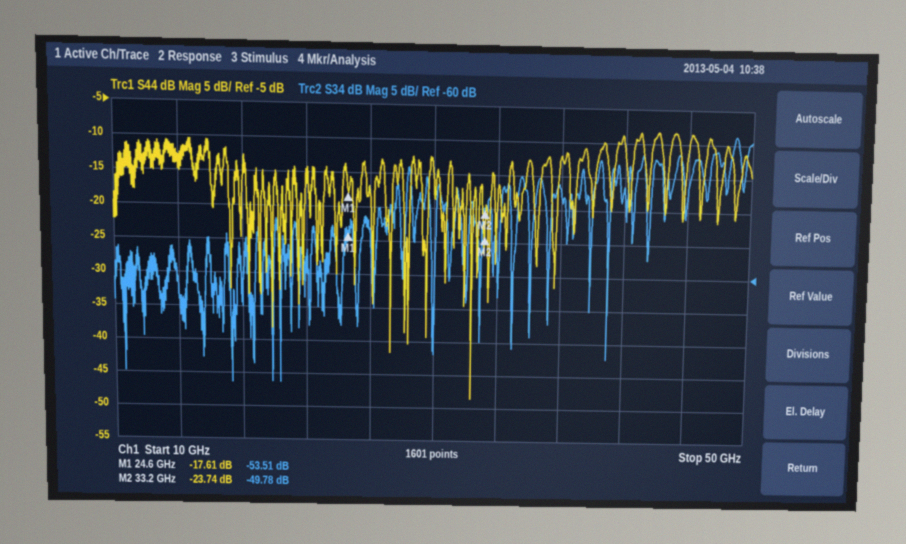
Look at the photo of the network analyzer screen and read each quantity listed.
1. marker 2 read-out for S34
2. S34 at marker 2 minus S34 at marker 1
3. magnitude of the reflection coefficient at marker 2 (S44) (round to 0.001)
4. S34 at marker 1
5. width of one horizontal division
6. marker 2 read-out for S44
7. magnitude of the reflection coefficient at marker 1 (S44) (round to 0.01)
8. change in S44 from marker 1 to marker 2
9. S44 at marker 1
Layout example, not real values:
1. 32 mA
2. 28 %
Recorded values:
1. -49.78 dB
2. 3.73 dB
3. 0.065
4. -53.51 dB
5. 4 GHz
6. -23.74 dB
7. 0.13
8. -6.13 dB
9. -17.61 dB
